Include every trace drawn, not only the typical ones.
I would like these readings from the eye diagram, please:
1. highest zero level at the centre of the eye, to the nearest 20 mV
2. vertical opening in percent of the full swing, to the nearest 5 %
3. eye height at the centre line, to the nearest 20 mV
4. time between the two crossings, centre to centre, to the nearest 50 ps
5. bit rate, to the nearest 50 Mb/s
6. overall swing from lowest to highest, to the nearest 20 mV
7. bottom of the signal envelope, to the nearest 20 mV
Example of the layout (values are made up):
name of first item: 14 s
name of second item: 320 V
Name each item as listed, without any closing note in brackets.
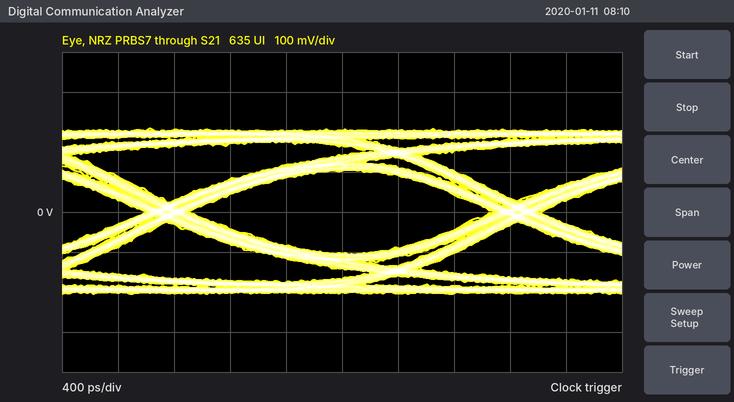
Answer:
highest zero level at the centre of the eye, to the nearest 20 mV: -100 mV
vertical opening in percent of the full swing, to the nearest 5 %: 50 %
eye height at the centre line, to the nearest 20 mV: 200 mV
time between the two crossings, centre to centre, to the nearest 50 ps: 2.50 ns
bit rate, to the nearest 50 Mb/s: 400 Mb/s
overall swing from lowest to highest, to the nearest 20 mV: 420 mV
bottom of the signal envelope, to the nearest 20 mV: -200 mV
